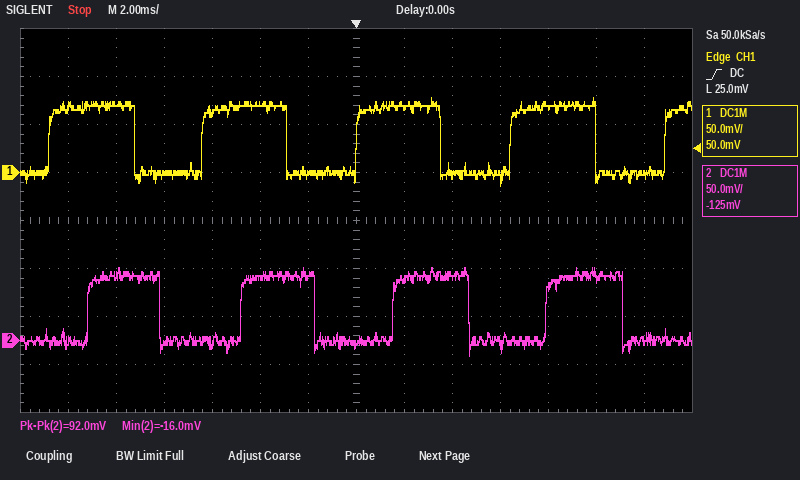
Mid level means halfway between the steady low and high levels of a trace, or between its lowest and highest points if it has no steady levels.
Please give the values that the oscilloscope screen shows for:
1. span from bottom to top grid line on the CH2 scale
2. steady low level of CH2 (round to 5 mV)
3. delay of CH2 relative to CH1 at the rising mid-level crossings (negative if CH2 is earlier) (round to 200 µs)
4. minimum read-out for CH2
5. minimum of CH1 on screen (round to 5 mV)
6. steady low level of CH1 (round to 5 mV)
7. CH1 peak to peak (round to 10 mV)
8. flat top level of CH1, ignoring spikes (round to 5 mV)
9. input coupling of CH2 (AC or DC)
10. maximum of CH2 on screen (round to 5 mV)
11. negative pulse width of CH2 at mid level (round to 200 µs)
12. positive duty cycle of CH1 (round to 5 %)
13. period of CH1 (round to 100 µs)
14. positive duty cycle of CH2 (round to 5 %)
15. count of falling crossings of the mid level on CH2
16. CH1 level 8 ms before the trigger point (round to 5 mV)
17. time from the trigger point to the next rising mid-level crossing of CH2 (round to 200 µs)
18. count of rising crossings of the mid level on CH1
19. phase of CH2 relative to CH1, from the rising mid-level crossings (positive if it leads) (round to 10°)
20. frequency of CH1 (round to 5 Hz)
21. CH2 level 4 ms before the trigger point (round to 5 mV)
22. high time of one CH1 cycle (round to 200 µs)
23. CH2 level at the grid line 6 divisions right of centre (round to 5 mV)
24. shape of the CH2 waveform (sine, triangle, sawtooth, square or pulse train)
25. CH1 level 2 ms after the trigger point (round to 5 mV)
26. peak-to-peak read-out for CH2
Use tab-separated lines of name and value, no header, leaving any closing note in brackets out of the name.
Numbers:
span from bottom to top grid line on the CH2 scale	400 mV
steady low level of CH2	0 mV
delay of CH2 relative to CH1 at the rising mid-level crossings (negative if CH2 is earlier)	+1.6 ms
minimum read-out for CH2	-16.0 mV
minimum of CH1 on screen	-15 mV
steady low level of CH1	0 mV
CH1 peak to peak	90 mV
flat top level of CH1, ignoring spikes	70 mV
input coupling of CH2	DC
maximum of CH2 on screen	75 mV
negative pulse width of CH2 at mid level	3.2 ms
positive duty cycle of CH1	55 %
period of CH1	6.4 ms
positive duty cycle of CH2	50 %
count of falling crossings of the mid level on CH2	4
CH1 level 8 ms before the trigger point	0 mV
time from the trigger point to the next rising mid-level crossing of CH2	1.6 ms
count of rising crossings of the mid level on CH1	5
phase of CH2 relative to CH1, from the rising mid-level crossings (positive if it leads)	-90°
frequency of CH1	155 Hz
CH2 level 4 ms before the trigger point	65 mV
high time of one CH1 cycle	3.6 ms
CH2 level at the grid line 6 divisions right of centre	0 mV
shape of the CH2 waveform	square
CH1 level 2 ms after the trigger point	70 mV
peak-to-peak read-out for CH2	92.0 mV
